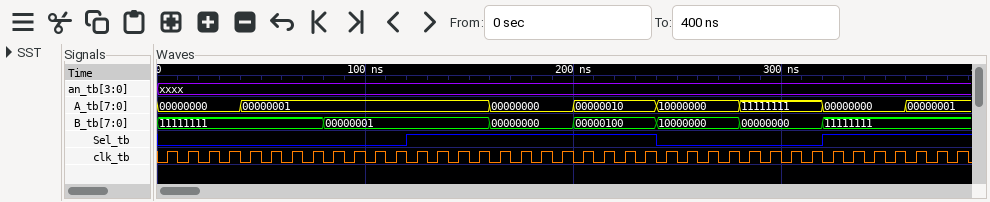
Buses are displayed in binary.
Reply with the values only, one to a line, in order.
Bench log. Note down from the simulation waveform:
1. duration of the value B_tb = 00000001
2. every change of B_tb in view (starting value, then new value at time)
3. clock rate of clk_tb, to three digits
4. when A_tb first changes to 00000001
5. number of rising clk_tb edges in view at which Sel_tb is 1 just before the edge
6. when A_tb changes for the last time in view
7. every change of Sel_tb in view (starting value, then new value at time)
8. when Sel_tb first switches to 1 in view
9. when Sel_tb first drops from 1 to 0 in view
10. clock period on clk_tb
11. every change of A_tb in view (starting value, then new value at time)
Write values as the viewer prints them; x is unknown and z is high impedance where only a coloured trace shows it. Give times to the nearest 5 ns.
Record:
80 ns
11111111, 00000001 at 80 ns, 00000000 at 160 ns, 00000100 at 200 ns, 10000000 at 240 ns, 00000000 at 280 ns, 11111111 at 320 ns
100 MHz
40 ns
19
360 ns
0, 1 at 120 ns, 0 at 240 ns, 1 at 320 ns
120 ns
240 ns
10 ns
00000000, 00000001 at 40 ns, 00000000 at 160 ns, 00000010 at 200 ns, 10000000 at 240 ns, 11111111 at 280 ns, 00000000 at 320 ns, 00000001 at 360 ns
